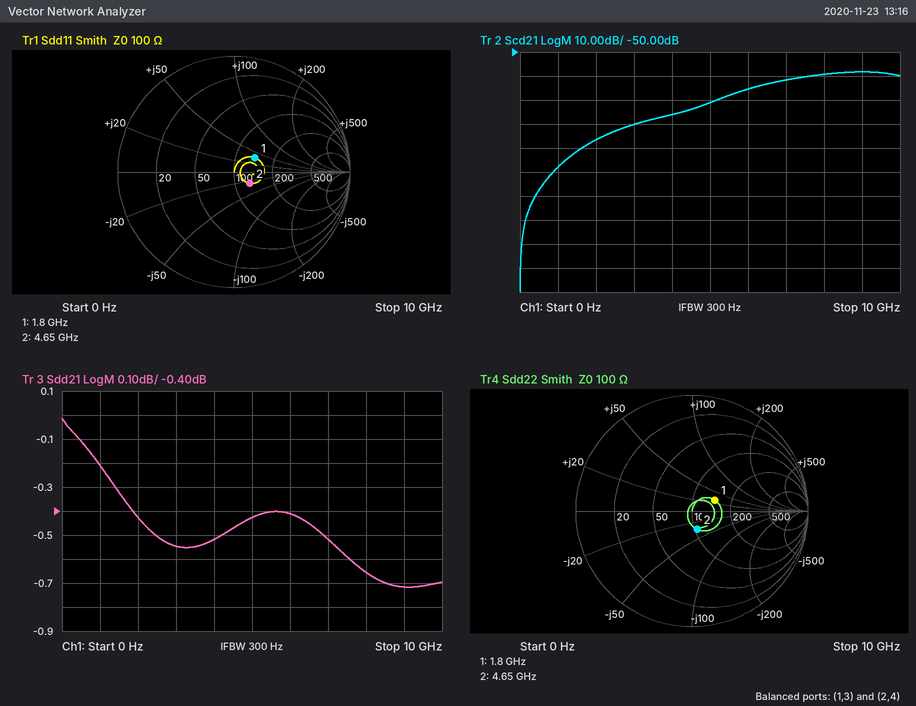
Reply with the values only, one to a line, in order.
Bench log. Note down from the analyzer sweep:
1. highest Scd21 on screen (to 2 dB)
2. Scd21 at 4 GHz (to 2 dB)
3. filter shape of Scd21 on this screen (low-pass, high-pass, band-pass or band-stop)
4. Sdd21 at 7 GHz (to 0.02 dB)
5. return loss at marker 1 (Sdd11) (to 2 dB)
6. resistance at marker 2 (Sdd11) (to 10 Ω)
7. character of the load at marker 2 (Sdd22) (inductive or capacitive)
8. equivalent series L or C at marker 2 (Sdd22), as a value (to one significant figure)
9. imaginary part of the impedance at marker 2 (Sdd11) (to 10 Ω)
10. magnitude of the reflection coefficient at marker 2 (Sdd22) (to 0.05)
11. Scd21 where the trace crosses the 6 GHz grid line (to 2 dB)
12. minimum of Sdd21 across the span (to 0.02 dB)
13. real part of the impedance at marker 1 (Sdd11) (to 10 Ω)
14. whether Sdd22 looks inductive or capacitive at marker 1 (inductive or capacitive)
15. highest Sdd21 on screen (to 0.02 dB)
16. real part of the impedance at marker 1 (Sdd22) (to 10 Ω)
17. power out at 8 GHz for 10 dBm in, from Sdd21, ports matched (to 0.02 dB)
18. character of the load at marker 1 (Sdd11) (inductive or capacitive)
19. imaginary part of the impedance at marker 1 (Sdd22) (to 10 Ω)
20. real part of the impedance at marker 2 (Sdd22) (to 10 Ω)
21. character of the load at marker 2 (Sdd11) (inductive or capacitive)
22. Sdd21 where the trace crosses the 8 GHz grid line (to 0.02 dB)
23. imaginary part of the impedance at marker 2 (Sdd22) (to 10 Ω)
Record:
-58 dB
-76 dB
high-pass
-0.52 dB
14 dB
130 Ω
capacitive
1 pF
-30 Ω
0.15
-66 dB
-0.72 dB
140 Ω
inductive
-0.02 dB
150 Ω
9.34 dBm
inductive
+30 Ω
100 Ω
capacitive
-0.66 dB
-30 Ω
